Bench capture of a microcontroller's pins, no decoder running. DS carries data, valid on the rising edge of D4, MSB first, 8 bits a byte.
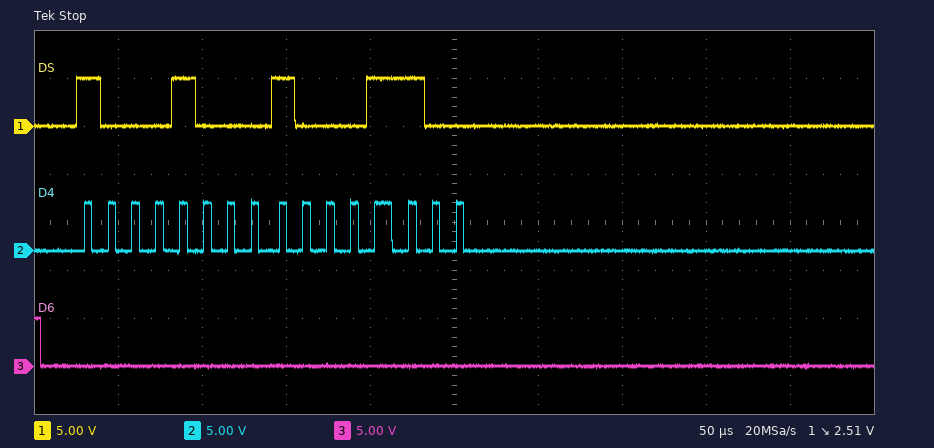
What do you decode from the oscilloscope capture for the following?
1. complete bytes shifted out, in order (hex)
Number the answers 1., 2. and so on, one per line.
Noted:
1. 0x88 0x8C
